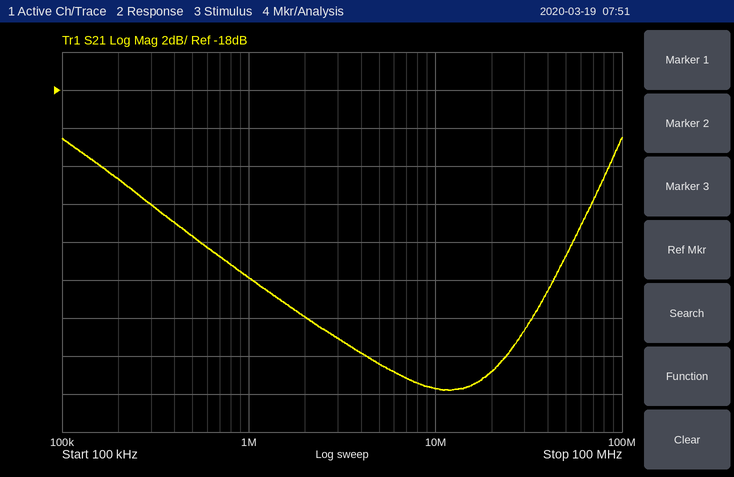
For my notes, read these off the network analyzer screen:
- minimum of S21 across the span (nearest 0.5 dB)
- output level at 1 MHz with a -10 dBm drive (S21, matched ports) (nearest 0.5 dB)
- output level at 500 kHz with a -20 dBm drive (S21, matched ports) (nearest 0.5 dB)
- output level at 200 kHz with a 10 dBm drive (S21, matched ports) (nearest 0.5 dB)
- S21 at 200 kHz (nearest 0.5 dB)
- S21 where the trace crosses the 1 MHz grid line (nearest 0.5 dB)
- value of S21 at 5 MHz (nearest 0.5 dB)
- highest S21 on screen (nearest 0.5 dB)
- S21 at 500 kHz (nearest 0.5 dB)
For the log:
-34.0 dB
-38.0 dBm
-45.5 dBm
-12.5 dBm
-22.5 dB
-28.0 dB
-32.5 dB
-20.5 dB
-25.5 dB
